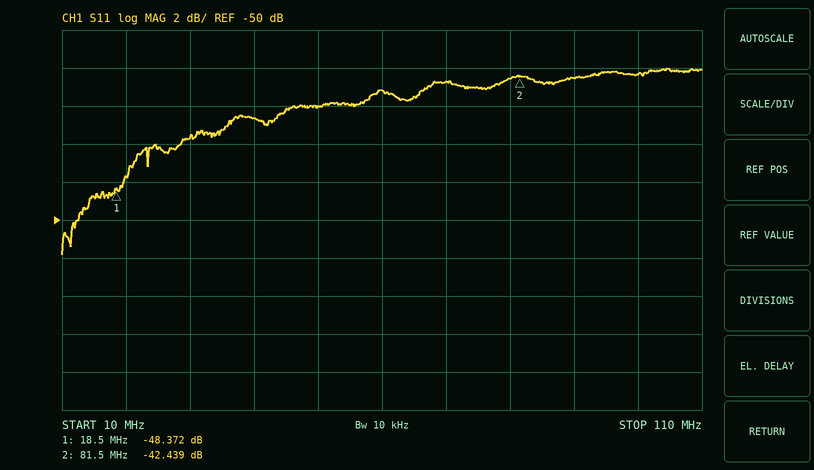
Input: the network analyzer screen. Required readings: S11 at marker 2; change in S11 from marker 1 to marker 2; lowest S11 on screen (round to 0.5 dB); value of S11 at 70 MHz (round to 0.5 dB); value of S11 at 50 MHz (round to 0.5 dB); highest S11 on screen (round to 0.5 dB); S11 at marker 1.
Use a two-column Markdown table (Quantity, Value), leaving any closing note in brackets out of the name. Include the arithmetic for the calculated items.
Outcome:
| Quantity | Value |
|---|---|
| S11 at marker 2 | -42.439 dB |
| change in S11 from marker 1 to marker 2 | -42.439 − (-48.372) = 5.933 dB |
| lowest S11 on screen | -52.0 dB |
| value of S11 at 70 MHz | -42.5 dB |
| value of S11 at 50 MHz | -44.0 dB |
| highest S11 on screen | -42.0 dB |
| S11 at marker 1 | -48.372 dB |
